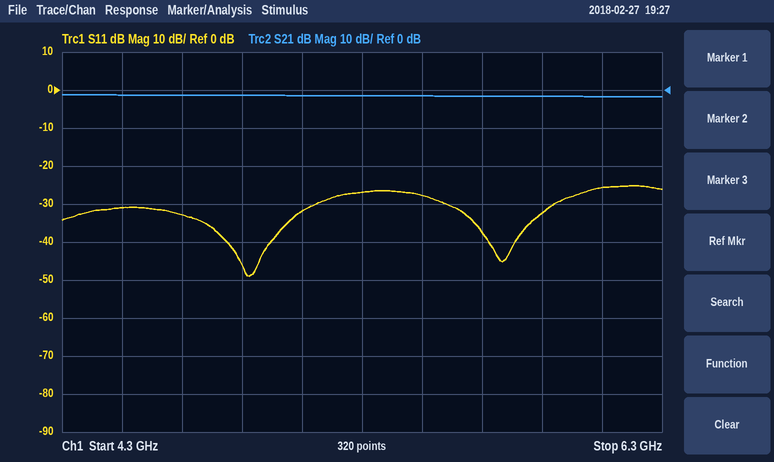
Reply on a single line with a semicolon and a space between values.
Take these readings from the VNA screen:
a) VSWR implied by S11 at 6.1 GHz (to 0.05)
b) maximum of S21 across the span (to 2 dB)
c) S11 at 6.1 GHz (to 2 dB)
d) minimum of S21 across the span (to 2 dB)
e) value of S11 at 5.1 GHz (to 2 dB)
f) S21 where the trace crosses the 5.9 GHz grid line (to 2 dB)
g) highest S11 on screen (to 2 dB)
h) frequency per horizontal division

1.10; -2 dB; -26 dB; -2 dB; -32 dB; -2 dB; -26 dB; 200 MHz
